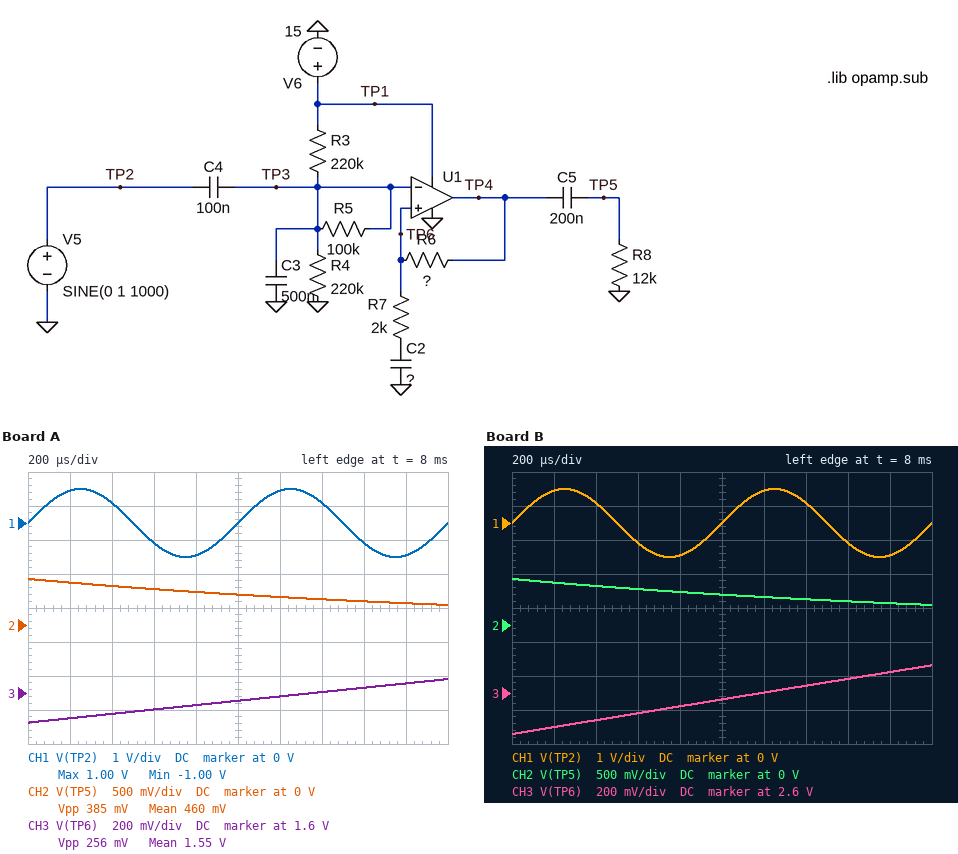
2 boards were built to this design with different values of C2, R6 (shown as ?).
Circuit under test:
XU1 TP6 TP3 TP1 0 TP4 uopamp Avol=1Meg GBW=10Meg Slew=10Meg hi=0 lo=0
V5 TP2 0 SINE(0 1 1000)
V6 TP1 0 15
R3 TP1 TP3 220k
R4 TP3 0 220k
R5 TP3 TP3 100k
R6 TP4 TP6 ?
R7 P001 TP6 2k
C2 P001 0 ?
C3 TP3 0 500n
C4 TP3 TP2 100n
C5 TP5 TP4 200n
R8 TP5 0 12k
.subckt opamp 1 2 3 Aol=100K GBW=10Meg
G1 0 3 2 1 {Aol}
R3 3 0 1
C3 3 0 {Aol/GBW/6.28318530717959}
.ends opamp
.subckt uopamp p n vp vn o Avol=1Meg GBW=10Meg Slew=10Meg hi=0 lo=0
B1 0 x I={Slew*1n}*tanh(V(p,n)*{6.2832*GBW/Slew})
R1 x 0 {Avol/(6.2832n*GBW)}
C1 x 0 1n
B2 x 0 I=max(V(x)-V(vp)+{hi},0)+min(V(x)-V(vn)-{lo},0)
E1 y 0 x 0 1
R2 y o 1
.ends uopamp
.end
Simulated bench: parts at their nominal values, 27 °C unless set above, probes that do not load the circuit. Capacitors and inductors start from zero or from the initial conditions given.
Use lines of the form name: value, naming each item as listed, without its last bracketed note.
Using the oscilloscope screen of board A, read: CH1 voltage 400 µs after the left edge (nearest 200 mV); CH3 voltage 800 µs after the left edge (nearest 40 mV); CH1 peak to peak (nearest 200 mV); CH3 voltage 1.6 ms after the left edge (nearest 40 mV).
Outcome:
CH1 voltage 400 µs after the left edge: 600 mV
CH3 voltage 800 µs after the left edge: 1.52 V
CH1 peak to peak: 2.0 V
CH3 voltage 1.6 ms after the left edge: 1.64 V
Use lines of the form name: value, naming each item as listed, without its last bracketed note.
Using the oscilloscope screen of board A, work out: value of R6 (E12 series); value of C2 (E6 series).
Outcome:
value of R6: 68 kΩ
value of C2: 1.5 µF
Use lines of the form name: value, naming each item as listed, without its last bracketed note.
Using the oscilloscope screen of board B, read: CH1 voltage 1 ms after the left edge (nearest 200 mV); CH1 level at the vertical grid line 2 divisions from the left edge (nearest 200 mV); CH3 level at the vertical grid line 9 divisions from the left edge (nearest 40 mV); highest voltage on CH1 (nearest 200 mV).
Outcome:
CH1 voltage 1 ms after the left edge: 0 V
CH1 level at the vertical grid line 2 divisions from the left edge: 600 mV
CH3 level at the vertical grid line 9 divisions from the left edge: 2.72 V
highest voltage on CH1: 1.0 V
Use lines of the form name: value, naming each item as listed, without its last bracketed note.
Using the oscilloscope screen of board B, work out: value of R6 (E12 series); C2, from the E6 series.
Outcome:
value of R6: 39 kΩ
C2, from the E6 series: 1.5 µF
